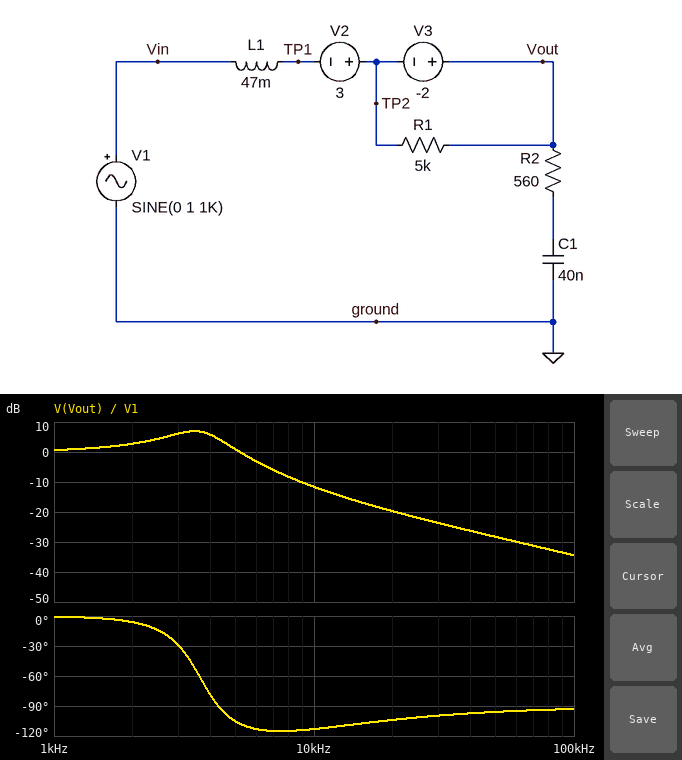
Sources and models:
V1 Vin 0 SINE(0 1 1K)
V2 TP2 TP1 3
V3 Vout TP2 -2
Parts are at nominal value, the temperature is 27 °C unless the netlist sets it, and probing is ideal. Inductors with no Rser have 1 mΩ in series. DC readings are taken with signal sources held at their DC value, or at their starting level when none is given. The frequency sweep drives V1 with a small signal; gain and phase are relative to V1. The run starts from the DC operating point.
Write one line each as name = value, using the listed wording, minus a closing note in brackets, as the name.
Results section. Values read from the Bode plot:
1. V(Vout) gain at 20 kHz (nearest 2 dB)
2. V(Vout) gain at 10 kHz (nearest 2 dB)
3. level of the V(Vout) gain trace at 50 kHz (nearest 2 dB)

V(Vout) gain at 20 kHz = -20 dB
V(Vout) gain at 10 kHz = -12 dB
level of the V(Vout) gain trace at 50 kHz = -28 dB
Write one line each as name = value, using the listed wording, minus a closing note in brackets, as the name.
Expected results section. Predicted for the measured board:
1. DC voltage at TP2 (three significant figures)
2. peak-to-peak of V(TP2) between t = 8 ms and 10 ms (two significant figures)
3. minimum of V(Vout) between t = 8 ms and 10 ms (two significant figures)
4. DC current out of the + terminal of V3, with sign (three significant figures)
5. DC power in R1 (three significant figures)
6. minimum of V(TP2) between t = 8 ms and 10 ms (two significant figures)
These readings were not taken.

DC voltage at TP2 = 3.00 V
peak-to-peak of V(TP2) between t = 8 ms and 10 ms = 2.2 V
minimum of V(Vout) between t = 8 ms and 10 ms = -78 mV
DC current out of the + terminal of V3, with sign = -400 µA
DC power in R1 = 800 µW
minimum of V(TP2) between t = 8 ms and 10 ms = 1.9 V
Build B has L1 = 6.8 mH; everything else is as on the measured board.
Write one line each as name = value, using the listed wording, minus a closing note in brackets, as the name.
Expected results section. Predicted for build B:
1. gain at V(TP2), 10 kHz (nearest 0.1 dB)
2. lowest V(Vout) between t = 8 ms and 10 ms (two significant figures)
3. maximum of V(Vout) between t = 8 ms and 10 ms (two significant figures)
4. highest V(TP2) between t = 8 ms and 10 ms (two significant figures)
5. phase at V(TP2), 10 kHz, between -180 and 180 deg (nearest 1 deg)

gain at V(TP2), 10 kHz = 1.8 dB
lowest V(Vout) between t = 8 ms and 10 ms = -11 mV
maximum of V(Vout) between t = 8 ms and 10 ms = 2.0 V
highest V(TP2) between t = 8 ms and 10 ms = 4.0 V
phase at V(TP2), 10 kHz, between -180 and 180 deg = -38 deg
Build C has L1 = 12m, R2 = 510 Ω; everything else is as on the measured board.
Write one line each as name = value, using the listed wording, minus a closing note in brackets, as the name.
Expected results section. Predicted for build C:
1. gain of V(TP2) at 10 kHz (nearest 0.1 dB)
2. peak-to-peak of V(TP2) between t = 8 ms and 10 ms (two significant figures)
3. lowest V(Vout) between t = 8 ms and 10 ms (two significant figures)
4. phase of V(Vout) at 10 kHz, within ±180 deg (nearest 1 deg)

gain of V(TP2) at 10 kHz = 0.3 dB
peak-to-peak of V(TP2) between t = 8 ms and 10 ms = 2.0 V
lowest V(Vout) between t = 8 ms and 10 ms = -19 mV
phase of V(Vout) at 10 kHz, within ±180 deg = -73 deg
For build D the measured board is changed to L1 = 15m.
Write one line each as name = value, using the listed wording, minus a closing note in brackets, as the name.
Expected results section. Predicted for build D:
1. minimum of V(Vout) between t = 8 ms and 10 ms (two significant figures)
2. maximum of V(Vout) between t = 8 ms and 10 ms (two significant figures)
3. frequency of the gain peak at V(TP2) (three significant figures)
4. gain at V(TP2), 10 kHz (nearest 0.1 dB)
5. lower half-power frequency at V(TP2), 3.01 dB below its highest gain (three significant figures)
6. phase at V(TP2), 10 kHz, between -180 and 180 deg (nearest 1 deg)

minimum of V(Vout) between t = 8 ms and 10 ms = -24 mV
maximum of V(Vout) between t = 8 ms and 10 ms = 2.0 V
frequency of the gain peak at V(TP2) = 5.66 kHz
gain at V(TP2), 10 kHz = -1.1 dB
lower half-power frequency at V(TP2), 3.01 dB below its highest gain = 1.90 kHz
phase at V(TP2), 10 kHz, between -180 and 180 deg = -80 deg
